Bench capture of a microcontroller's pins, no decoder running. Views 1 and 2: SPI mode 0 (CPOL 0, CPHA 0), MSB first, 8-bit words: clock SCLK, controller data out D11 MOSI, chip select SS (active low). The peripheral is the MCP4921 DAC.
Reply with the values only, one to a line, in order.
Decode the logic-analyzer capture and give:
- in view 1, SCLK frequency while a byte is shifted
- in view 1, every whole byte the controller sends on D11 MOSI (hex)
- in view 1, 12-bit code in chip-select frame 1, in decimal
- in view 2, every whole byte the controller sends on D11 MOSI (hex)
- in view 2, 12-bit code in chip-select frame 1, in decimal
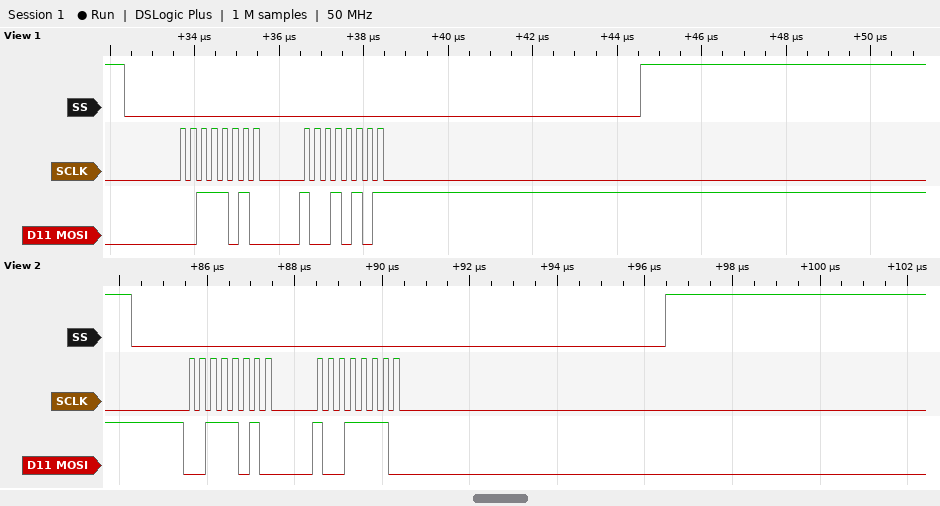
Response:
4 MHz
3A 95
2709
3A 9E
2718
